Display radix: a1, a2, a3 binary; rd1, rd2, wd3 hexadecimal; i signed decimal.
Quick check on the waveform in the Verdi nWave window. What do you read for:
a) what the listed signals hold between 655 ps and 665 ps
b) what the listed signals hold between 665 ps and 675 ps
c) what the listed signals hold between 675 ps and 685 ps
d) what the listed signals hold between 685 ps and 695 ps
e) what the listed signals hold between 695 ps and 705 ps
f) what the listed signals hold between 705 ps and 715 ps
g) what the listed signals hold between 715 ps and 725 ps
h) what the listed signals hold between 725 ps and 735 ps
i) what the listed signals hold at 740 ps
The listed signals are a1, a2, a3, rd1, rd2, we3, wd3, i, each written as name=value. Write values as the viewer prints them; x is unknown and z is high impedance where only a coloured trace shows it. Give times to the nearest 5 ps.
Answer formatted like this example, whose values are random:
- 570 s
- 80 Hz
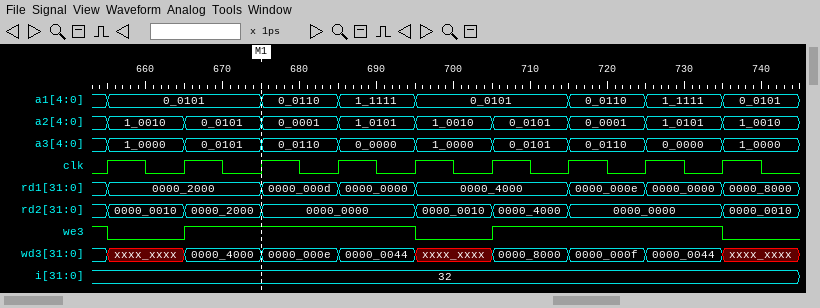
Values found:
- a1=0_0101, a2=1_0010, a3=1_0000, rd1=0000_2000, rd2=0000_0010, we3=0, wd3=xxxx_xxxx, i=32
- a1=0_0101, a2=0_0101, a3=0_0101, rd1=0000_2000, rd2=0000_2000, we3=1, wd3=0000_4000, i=32
- a1=0_0110, a2=0_0001, a3=0_0110, rd1=0000_000d, rd2=0000_0000, we3=1, wd3=0000_000e, i=32
- a1=1_1111, a2=1_0101, a3=0_0000, rd1=0000_0000, rd2=0000_0000, we3=1, wd3=0000_0044, i=32
- a1=0_0101, a2=1_0010, a3=1_0000, rd1=0000_4000, rd2=0000_0010, we3=0, wd3=xxxx_xxxx, i=32
- a1=0_0101, a2=0_0101, a3=0_0101, rd1=0000_4000, rd2=0000_4000, we3=1, wd3=0000_8000, i=32
- a1=0_0110, a2=0_0001, a3=0_0110, rd1=0000_000e, rd2=0000_0000, we3=1, wd3=0000_000f, i=32
- a1=1_1111, a2=1_0101, a3=0_0000, rd1=0000_0000, rd2=0000_0000, we3=1, wd3=0000_0044, i=32
- a1=0_0101, a2=1_0010, a3=1_0000, rd1=0000_8000, rd2=0000_0010, we3=0, wd3=xxxx_xxxx, i=32
